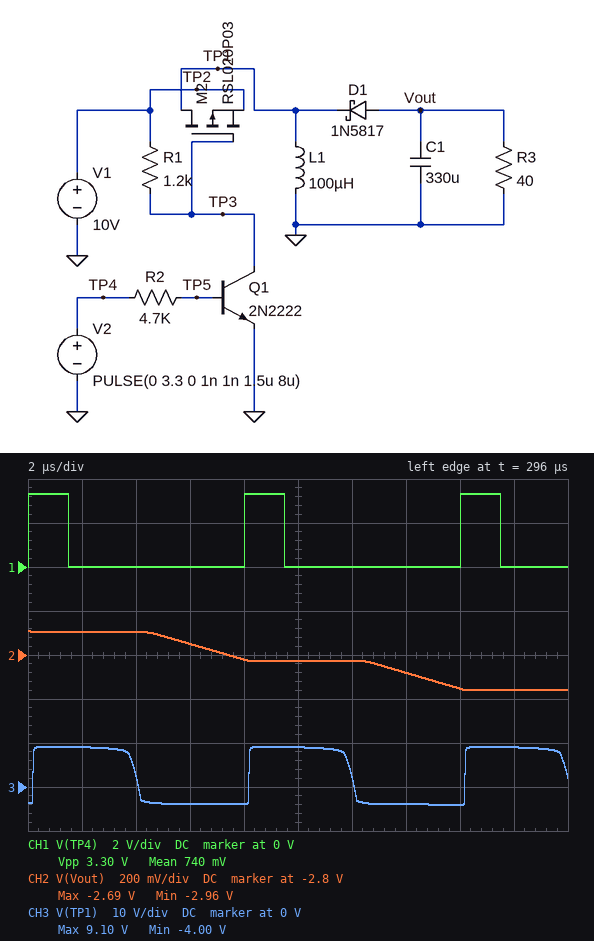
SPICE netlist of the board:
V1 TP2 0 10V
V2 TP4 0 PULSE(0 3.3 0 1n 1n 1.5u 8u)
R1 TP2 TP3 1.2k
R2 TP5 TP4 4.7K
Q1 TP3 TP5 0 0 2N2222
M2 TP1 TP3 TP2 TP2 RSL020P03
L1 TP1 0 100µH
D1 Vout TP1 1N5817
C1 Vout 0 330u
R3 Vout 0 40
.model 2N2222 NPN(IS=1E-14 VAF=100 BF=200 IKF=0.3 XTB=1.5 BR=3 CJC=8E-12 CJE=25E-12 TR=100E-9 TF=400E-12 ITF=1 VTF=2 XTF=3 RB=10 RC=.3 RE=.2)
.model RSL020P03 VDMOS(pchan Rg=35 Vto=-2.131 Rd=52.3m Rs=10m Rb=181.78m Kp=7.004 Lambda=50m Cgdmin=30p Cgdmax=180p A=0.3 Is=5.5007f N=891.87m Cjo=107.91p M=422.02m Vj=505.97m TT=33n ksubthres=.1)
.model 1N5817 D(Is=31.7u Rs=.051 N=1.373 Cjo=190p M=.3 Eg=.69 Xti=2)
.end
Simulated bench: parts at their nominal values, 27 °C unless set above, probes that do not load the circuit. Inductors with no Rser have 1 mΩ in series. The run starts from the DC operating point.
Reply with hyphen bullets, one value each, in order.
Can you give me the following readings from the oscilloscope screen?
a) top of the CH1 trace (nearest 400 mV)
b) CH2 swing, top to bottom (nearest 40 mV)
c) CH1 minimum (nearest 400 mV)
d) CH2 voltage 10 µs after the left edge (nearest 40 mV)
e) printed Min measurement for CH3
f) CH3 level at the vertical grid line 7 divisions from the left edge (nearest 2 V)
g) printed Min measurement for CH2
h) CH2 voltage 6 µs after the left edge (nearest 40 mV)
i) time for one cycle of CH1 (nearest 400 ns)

- 3.2 V
- 280 mV
- 0 V
- -2.84 V
- -4.00 V
- -4 V
- -2.96 V
- -2.76 V
- 8.0 µs
